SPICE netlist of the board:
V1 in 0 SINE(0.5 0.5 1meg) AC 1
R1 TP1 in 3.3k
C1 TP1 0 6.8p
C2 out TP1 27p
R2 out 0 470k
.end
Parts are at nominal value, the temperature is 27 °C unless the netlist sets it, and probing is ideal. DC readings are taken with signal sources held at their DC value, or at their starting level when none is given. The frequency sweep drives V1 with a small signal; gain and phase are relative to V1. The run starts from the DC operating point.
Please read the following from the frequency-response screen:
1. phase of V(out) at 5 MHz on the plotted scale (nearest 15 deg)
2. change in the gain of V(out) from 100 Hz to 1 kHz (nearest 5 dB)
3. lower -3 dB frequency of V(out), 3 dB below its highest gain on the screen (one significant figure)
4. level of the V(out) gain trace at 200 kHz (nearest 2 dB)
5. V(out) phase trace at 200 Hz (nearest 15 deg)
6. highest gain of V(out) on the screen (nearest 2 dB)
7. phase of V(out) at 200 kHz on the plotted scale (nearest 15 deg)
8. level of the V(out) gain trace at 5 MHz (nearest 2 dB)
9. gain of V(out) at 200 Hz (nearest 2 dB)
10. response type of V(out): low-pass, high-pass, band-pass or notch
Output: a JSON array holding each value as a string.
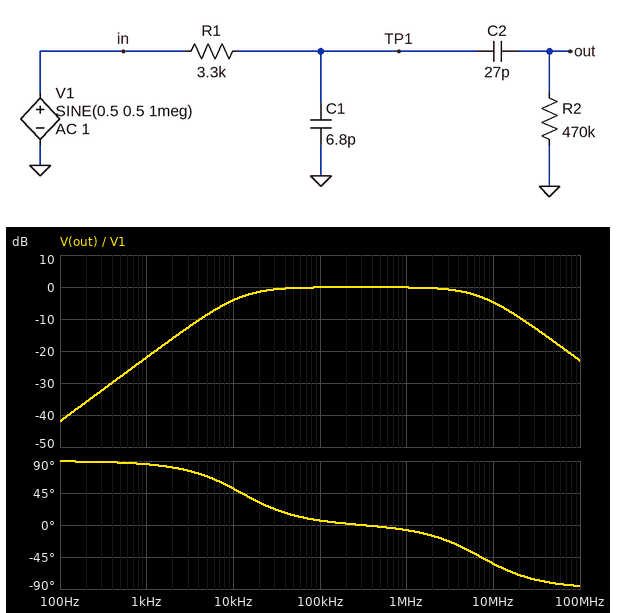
["-30 deg", "20 dB", "10 kHz", "0 dB", "90 deg", "0 dB", "0 deg", "-2 dB", "-36 dB", "band-pass"]
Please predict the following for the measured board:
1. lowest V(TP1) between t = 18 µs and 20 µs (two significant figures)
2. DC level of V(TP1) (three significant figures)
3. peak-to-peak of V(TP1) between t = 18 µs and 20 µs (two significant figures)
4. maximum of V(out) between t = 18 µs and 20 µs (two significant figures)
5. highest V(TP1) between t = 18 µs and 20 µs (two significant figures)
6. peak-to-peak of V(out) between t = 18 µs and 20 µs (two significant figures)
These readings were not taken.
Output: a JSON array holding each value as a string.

["8.3 mV", "500 mV", "980 mV", "490 mV", "990 mV", "980 mV"]
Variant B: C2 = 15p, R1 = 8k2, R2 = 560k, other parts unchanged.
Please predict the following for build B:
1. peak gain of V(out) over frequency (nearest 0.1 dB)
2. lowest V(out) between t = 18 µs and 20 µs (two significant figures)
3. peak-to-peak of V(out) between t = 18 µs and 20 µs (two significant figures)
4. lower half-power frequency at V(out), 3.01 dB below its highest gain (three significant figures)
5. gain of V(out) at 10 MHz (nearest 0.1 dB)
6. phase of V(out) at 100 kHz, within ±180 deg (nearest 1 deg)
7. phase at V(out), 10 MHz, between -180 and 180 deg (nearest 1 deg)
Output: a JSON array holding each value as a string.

["-0.2 dB", "-470 mV", "930 mV", "18.4 kHz", "-11.2 dB", "9 deg", "-74 deg"]
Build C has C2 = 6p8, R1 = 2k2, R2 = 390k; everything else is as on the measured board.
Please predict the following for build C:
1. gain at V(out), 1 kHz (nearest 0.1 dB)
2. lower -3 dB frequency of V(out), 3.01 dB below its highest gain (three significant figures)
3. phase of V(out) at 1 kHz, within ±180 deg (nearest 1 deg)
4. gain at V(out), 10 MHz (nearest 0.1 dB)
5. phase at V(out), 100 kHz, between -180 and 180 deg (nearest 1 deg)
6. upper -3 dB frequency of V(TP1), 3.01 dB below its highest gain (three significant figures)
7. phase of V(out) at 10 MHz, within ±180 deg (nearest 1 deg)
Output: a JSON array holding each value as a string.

["-35.6 dB", "59.0 kHz", "89 deg", "-2.8 dB", "30 deg", "10.6 MHz", "-43 deg"]
